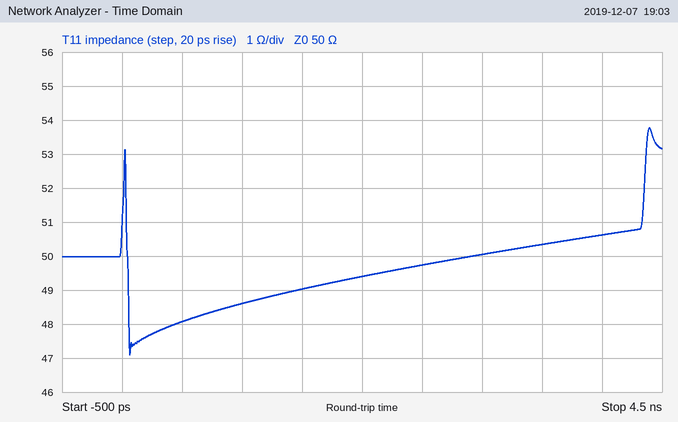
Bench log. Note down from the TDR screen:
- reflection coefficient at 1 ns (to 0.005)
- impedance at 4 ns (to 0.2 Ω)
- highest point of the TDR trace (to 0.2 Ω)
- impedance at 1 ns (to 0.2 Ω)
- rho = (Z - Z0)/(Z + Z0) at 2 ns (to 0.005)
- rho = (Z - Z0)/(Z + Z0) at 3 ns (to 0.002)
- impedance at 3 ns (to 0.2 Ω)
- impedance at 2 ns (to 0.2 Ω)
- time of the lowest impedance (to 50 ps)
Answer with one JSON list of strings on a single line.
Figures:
["-0.015", "50.6 Ω", "53.8 Ω", "48.6 Ω", "-0.005", "0.000", "50.0 Ω", "49.4 Ω", "50 ps"]
